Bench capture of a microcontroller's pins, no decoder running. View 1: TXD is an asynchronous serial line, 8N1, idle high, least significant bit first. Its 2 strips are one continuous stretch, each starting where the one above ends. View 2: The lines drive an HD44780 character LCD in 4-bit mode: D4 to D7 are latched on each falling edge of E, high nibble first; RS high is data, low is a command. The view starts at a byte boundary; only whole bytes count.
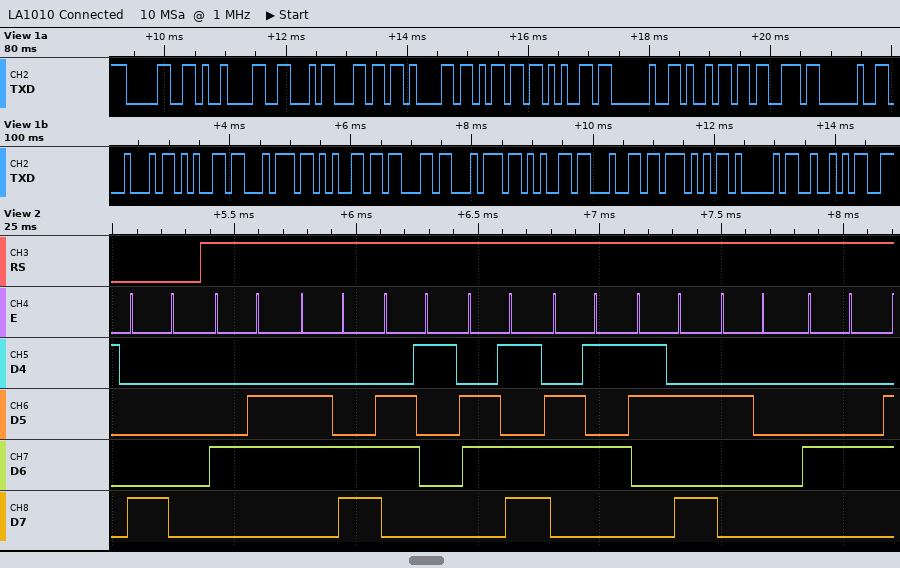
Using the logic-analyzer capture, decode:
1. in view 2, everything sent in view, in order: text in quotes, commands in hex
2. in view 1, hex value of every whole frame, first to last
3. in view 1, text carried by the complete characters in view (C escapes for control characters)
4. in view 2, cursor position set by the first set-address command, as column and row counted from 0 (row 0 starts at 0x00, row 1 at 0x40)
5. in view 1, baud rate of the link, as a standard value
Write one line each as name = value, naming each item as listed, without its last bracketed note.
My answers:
in view 2, everything sent in view, in order: text in quotes, commands in hex = 0x80 "Flame: D"
in view 1, hex value of every whole frame, first to last = 30 09 46 6C 61 6D 65 20 69 73 20 44 65 74 65 63 74 65 64 57 41 52
in view 1, text carried by the complete characters in view = "0\tFlame is DetectedWAR"
in view 2, cursor position set by the first set-address command, as column and row counted from 0 = column 0, row 0
in view 1, baud rate of the link, as a standard value = 9600 baud
